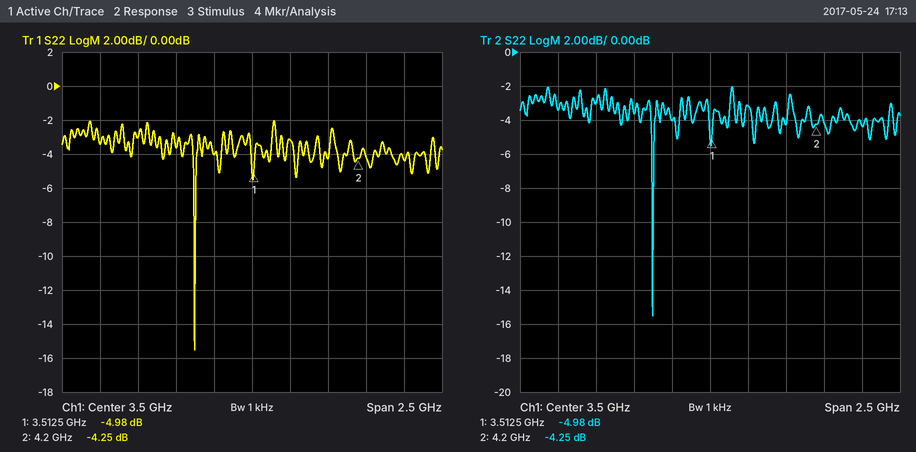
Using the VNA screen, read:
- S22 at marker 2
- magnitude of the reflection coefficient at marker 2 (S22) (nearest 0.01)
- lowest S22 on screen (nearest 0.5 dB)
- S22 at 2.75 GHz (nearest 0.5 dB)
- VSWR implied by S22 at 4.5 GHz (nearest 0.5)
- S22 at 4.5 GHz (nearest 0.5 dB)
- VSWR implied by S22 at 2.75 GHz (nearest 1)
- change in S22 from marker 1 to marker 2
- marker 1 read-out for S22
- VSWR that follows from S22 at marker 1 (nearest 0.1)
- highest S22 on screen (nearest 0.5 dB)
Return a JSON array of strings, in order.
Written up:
["-4.25 dB", "0.61", "-15.5 dB", "-3.0 dB", "4.0", "-4.5 dB", "6", "0.73 dB", "-4.98 dB", "3.6", "-2.0 dB"]
